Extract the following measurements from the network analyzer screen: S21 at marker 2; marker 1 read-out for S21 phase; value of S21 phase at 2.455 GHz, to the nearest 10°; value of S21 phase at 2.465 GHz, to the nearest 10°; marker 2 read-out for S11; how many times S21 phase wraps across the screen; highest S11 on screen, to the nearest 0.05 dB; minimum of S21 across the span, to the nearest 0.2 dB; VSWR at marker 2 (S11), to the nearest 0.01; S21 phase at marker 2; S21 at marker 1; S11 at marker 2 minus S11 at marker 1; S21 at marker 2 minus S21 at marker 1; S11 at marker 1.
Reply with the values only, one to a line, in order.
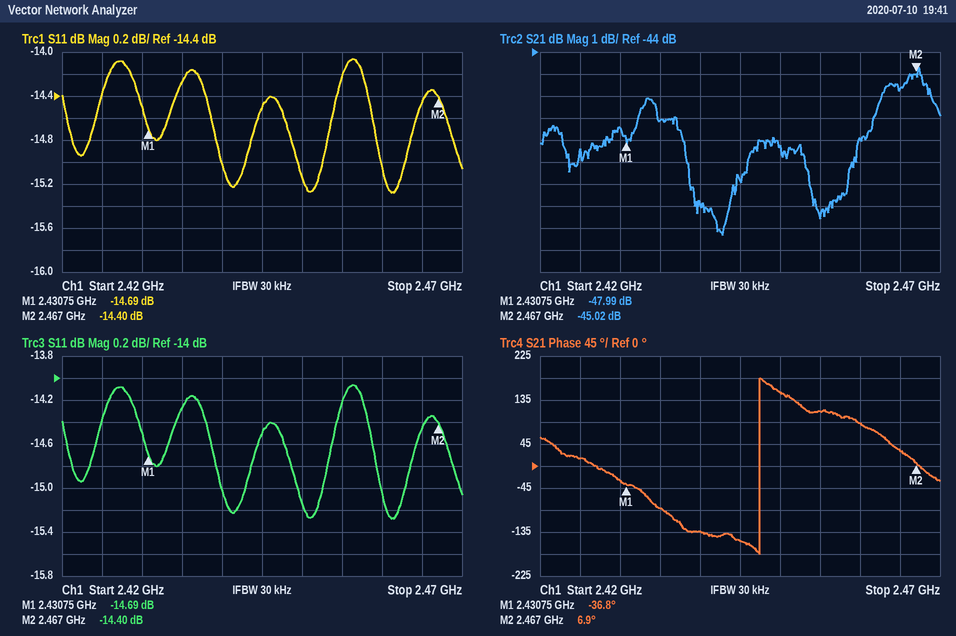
-45.02 dB
-36.8°
110°
30°
-14.40 dB
1
-14.05 dB
-52.4 dB
1.47
6.9°
-47.99 dB
0.29 dB
2.97 dB
-14.69 dB
